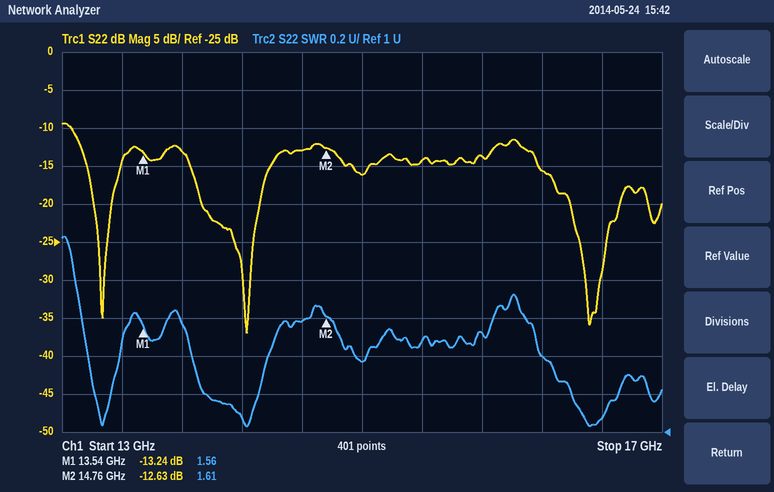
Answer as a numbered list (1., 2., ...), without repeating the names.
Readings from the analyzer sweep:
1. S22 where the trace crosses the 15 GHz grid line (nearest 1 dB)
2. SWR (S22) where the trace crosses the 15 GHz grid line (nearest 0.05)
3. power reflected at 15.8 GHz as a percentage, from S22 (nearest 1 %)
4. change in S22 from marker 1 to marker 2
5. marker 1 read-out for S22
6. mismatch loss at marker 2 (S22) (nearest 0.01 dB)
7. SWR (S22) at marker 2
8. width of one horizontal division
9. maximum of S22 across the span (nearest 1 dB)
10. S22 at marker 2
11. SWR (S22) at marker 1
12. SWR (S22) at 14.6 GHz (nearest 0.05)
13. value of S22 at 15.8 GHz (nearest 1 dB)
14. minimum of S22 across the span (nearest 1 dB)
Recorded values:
1. -16 dB
2. 1.35
3. 4 %
4. 0.61 dB
5. -13.24 dB
6. 0.24 dB
7. 1.61
8. 400 MHz
9. -9 dB
10. -12.63 dB
11. 1.56
12. 1.60
13. -14 dB
14. -37 dB
